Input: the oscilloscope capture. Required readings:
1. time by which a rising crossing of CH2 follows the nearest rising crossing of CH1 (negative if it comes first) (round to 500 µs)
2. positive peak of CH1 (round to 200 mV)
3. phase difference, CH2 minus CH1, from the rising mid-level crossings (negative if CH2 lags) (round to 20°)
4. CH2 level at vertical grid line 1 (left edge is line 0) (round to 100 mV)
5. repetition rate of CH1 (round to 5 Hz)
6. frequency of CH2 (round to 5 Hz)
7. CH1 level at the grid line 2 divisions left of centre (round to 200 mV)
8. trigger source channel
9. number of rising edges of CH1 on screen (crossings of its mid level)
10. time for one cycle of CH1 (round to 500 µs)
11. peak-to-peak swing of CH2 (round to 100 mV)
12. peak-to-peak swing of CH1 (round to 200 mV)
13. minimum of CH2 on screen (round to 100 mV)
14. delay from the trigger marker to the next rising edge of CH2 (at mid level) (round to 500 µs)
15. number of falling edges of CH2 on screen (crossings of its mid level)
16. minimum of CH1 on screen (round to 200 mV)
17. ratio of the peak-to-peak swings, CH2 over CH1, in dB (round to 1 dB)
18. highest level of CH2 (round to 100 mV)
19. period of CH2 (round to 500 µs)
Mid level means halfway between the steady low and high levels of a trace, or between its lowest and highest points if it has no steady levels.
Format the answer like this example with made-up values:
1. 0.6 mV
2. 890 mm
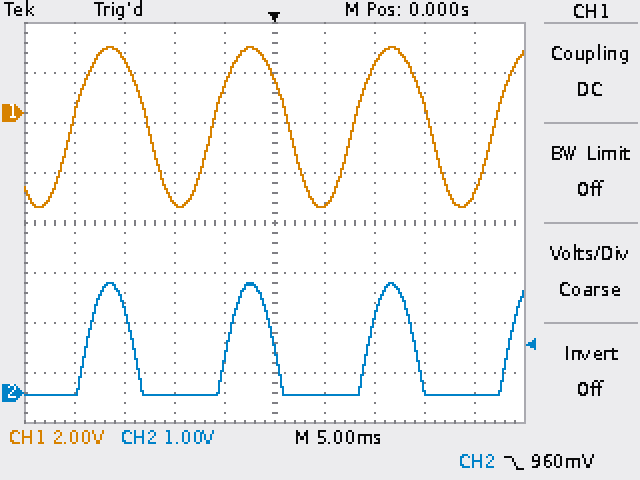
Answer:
1. +1.5 ms
2. 2.6 V
3. -40°
4. 0.0 V
5. 70 Hz
6. 70 Hz
7. -3.6 V
8. CH2
9. 4
10. 14.0 ms
11. 2.2 V
12. 6.4 V
13. 0.0 V
14. 9.5 ms
15. 3
16. -3.8 V
17. -9 dB
18. 2.2 V
19. 14.0 ms
